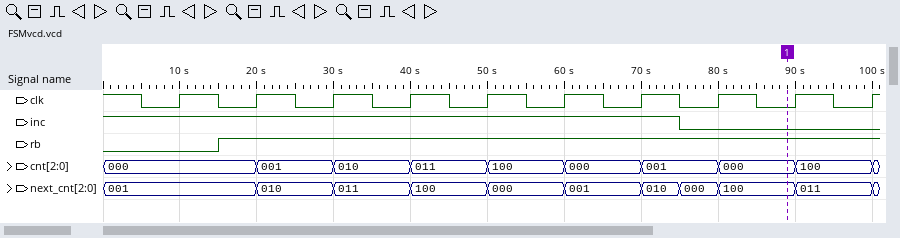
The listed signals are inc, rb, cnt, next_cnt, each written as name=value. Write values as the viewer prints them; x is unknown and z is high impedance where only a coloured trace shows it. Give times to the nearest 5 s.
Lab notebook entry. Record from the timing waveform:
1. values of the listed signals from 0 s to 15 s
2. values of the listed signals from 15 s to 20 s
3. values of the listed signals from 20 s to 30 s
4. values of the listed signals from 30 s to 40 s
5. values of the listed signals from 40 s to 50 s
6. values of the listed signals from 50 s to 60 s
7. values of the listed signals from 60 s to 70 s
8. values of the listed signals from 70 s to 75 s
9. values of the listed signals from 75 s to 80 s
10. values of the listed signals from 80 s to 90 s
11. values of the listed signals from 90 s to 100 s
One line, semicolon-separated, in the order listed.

inc=1, rb=0, cnt=000, next_cnt=001; inc=1, rb=1, cnt=000, next_cnt=001; inc=1, rb=1, cnt=001, next_cnt=010; inc=1, rb=1, cnt=010, next_cnt=011; inc=1, rb=1, cnt=011, next_cnt=100; inc=1, rb=1, cnt=100, next_cnt=000; inc=1, rb=1, cnt=000, next_cnt=001; inc=1, rb=1, cnt=001, next_cnt=010; inc=0, rb=1, cnt=001, next_cnt=000; inc=0, rb=1, cnt=000, next_cnt=100; inc=0, rb=1, cnt=100, next_cnt=011
